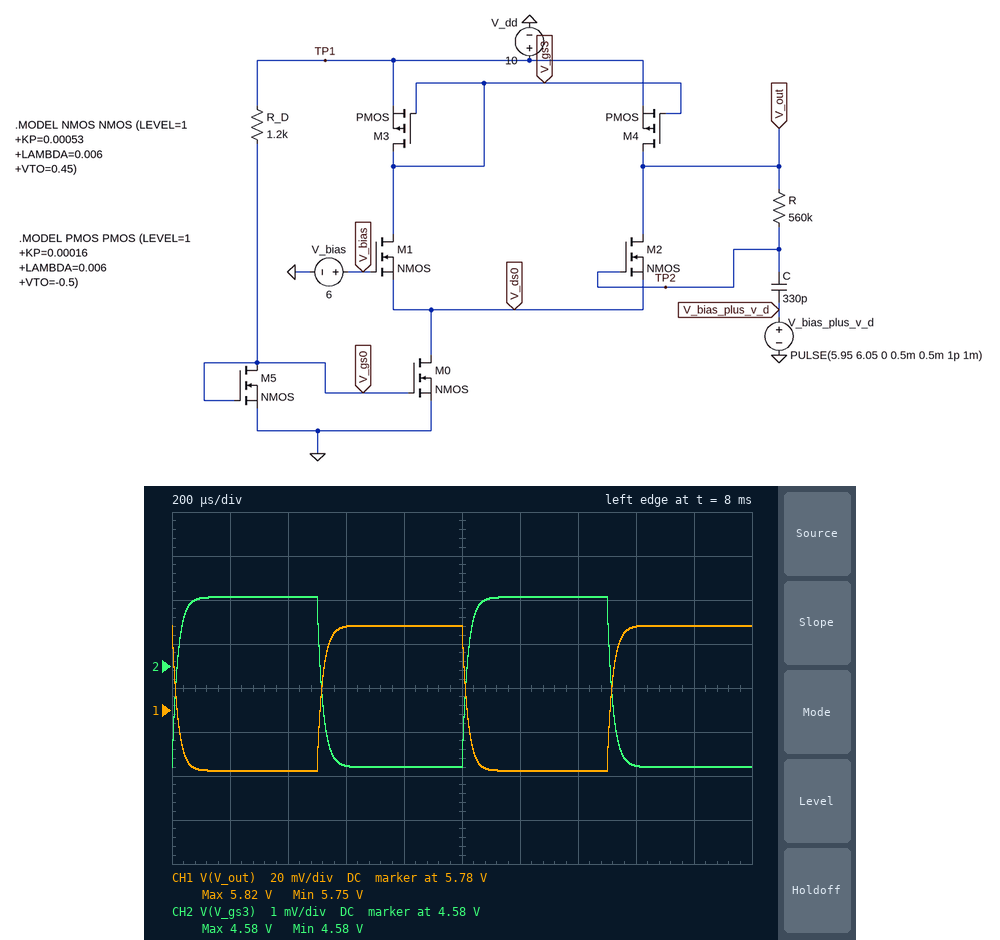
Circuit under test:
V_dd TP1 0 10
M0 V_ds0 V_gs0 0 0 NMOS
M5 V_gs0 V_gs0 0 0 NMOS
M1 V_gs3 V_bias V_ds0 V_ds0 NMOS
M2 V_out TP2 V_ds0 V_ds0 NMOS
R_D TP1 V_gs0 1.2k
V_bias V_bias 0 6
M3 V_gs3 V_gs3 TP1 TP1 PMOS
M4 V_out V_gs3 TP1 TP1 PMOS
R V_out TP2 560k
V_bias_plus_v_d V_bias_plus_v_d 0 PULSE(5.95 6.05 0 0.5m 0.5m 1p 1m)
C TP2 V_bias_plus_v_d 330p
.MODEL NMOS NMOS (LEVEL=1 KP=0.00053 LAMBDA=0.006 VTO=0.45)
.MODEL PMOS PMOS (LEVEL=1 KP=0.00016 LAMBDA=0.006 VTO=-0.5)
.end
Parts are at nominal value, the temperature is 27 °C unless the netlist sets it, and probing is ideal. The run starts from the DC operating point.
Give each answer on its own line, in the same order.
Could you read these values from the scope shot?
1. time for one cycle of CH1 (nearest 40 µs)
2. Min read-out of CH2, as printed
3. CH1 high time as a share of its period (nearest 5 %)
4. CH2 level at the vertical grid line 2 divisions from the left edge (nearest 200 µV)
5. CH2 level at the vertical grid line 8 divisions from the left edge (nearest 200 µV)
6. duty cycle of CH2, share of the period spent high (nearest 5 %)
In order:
1.00 ms
4.58 V
50 %
4.5816 V
4.5778 V
50 %
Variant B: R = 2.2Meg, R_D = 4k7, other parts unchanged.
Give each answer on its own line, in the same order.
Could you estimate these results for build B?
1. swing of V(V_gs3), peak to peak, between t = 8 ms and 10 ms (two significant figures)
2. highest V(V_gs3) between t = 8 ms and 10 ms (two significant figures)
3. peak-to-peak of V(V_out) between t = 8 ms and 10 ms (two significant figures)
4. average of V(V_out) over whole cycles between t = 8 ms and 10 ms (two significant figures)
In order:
1.4 mV
6.4 V
290 mV
6.0 V
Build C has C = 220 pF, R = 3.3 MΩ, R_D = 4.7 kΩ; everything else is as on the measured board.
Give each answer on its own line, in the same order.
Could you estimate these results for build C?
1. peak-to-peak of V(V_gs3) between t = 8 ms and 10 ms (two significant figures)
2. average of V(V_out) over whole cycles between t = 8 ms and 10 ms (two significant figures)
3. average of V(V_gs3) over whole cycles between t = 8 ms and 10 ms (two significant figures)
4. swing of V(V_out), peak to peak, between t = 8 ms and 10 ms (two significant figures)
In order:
1.4 mV
6.0 V
6.4 V
290 mV
